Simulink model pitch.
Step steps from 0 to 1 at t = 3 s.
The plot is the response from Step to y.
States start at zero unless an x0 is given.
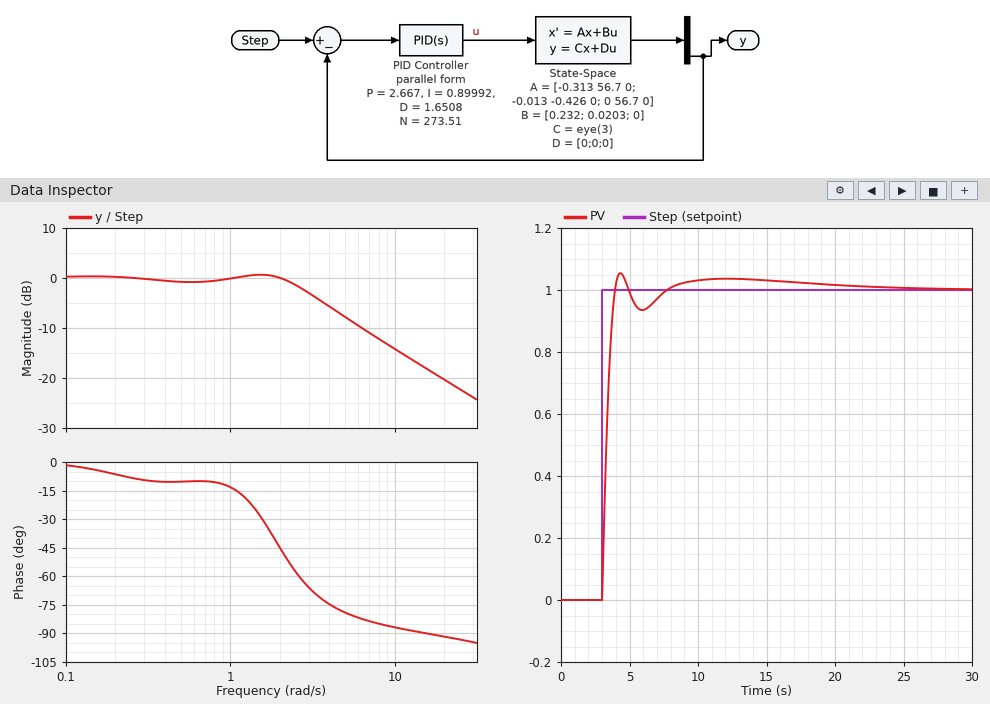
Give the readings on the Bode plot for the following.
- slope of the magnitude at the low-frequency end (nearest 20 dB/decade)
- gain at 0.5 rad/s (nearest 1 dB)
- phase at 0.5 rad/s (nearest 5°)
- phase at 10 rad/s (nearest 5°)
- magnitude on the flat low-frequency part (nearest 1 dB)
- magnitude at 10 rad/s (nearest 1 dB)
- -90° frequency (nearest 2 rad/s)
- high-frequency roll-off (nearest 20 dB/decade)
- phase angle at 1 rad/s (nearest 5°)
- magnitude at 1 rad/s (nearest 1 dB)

0 dB/decade
-1 dB
-10°
-85°
0 dB
-14 dB
16 rad/s
-20 dB/decade
-15°
0 dB
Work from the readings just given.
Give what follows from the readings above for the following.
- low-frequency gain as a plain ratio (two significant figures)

1.0
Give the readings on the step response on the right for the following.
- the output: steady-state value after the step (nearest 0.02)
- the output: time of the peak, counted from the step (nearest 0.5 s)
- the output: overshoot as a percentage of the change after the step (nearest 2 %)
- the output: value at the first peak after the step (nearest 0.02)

1.00
1.5 s
6 %
1.06
